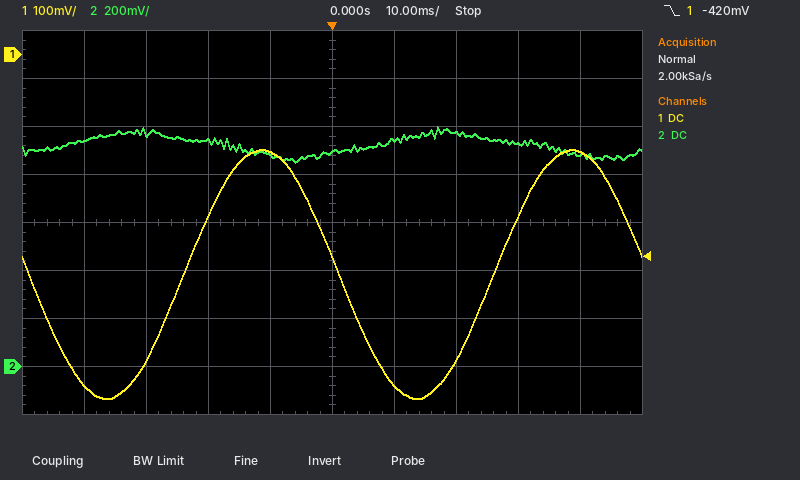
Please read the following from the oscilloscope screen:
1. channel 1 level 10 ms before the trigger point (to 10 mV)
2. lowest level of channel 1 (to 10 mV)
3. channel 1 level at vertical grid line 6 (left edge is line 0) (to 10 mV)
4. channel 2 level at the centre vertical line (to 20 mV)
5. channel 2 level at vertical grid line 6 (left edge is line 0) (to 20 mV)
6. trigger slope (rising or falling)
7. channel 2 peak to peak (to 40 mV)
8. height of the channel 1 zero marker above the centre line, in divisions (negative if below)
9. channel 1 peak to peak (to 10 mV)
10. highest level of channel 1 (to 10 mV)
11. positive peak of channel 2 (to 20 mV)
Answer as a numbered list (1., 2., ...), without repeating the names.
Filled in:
1. -200 mV
2. -720 mV
3. -690 mV
4. 900 mV
5. 940 mV
6. falling
7. 160 mV
8. +3.5 div
9. 520 mV
10. -200 mV
11. 1.00 V
